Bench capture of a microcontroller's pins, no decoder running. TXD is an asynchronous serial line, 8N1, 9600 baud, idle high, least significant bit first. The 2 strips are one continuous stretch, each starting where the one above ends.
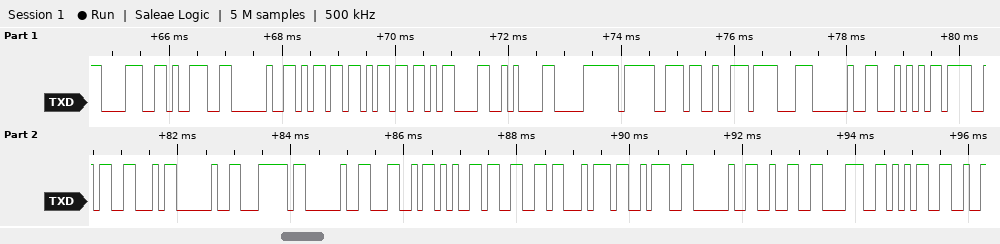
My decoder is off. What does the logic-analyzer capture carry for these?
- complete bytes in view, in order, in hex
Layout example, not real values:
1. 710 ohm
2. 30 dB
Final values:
1. 38 39 20 6D 6D 0D 0A F0 9F 93 8F 20 54 4F 46 20 7C 20 4C 65 66 74 3A 20 32 38 35
